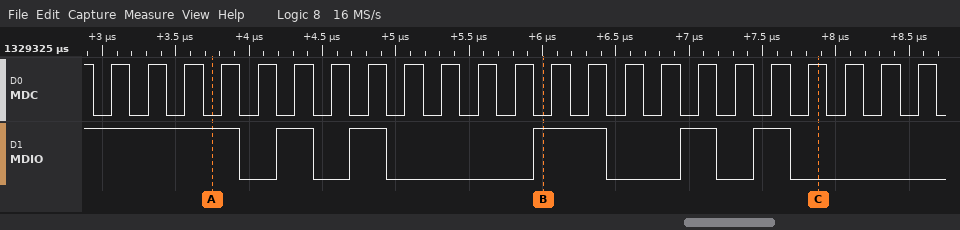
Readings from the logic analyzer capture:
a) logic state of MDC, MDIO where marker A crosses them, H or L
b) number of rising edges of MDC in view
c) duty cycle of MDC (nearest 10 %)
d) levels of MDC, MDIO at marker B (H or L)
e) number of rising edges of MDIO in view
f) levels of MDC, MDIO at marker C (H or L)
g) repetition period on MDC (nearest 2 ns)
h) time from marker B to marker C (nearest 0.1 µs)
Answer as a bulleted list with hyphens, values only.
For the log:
- MDC=L, MDIO=H
- 23
- 50 %
- MDC=L, MDIO=H
- 5
- MDC=H, MDIO=L
- 250 ns
- 1.9 µs
